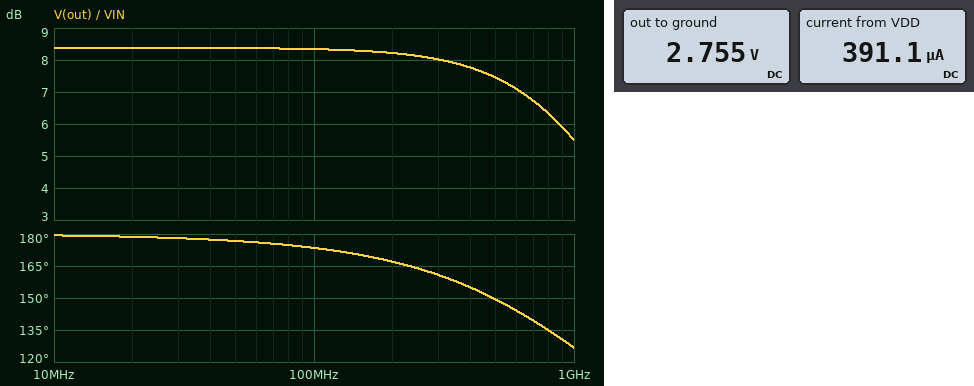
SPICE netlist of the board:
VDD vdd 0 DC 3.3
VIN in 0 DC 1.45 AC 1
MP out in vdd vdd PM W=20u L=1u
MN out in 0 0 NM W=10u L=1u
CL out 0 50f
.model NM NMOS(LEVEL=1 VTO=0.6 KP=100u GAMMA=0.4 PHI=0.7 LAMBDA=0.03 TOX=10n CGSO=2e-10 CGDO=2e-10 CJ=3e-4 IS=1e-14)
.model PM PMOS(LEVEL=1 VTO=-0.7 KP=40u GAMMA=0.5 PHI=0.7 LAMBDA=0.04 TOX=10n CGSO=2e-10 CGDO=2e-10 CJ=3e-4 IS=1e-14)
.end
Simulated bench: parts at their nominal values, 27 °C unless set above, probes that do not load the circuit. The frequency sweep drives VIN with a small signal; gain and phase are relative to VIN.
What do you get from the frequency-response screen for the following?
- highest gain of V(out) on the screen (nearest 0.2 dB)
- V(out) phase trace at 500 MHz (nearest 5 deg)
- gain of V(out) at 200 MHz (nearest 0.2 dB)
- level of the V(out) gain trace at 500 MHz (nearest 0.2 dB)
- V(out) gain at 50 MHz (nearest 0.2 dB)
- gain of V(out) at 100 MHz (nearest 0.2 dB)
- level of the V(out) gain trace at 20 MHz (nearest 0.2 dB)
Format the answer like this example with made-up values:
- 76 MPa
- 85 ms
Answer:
- 8.4 dB
- 150 deg
- 8.2 dB
- 7.4 dB
- 8.4 dB
- 8.4 dB
- 8.4 dB
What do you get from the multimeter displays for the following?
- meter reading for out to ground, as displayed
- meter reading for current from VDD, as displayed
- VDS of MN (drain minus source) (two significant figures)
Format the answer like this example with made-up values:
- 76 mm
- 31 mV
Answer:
- 2.755 V
- 391.1 µA
- 2.8 V
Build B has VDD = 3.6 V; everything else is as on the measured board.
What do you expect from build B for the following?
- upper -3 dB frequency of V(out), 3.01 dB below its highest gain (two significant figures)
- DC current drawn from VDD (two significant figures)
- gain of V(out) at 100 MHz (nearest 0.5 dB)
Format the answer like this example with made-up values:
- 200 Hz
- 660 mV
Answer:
- 1.8 GHz
- 400 µA
- 3.0 dB
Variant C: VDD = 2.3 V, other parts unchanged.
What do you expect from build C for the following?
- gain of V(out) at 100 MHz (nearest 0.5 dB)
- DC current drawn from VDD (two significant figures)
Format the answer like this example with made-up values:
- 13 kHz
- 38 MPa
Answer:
- -15.5 dB
- 9.8 µA
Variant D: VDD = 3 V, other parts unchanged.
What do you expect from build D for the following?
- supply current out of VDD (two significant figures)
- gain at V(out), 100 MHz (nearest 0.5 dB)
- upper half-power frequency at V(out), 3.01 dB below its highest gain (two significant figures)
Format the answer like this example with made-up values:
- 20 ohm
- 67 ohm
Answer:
- 320 µA
- 11.5 dB
- 810 MHz
